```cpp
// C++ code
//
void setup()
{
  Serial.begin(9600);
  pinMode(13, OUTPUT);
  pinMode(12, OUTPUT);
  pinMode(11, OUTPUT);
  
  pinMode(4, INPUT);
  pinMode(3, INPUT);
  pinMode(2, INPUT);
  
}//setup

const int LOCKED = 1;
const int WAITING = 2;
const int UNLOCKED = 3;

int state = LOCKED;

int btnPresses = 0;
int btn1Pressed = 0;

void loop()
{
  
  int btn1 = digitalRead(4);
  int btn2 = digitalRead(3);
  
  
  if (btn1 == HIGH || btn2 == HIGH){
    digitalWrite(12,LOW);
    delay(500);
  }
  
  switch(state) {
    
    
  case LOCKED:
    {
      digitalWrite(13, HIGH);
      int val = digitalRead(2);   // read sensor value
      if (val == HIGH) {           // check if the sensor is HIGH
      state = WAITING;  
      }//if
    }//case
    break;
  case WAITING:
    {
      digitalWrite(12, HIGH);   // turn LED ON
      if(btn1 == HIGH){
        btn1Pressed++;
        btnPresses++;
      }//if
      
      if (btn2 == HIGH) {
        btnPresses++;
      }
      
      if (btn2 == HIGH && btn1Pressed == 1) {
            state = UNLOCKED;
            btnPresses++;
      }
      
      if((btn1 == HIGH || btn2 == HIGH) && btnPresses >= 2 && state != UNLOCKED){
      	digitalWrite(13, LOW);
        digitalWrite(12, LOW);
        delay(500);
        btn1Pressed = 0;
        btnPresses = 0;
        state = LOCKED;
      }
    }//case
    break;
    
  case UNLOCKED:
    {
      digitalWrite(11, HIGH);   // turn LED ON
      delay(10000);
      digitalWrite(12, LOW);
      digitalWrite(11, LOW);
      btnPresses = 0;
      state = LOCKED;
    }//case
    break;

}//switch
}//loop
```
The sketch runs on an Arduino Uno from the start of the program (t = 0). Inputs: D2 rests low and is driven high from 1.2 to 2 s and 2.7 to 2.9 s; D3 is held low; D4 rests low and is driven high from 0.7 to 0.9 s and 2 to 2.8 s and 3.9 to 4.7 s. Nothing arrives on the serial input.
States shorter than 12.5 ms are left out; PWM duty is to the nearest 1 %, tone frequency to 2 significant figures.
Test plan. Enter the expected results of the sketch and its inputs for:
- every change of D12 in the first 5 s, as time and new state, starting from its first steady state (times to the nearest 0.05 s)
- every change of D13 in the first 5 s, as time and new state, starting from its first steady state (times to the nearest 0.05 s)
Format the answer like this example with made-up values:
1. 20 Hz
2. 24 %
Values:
1. 0 s low; 1.2 s high; 2 s low
2. 0 s high; 3 s low; 3.5 s high
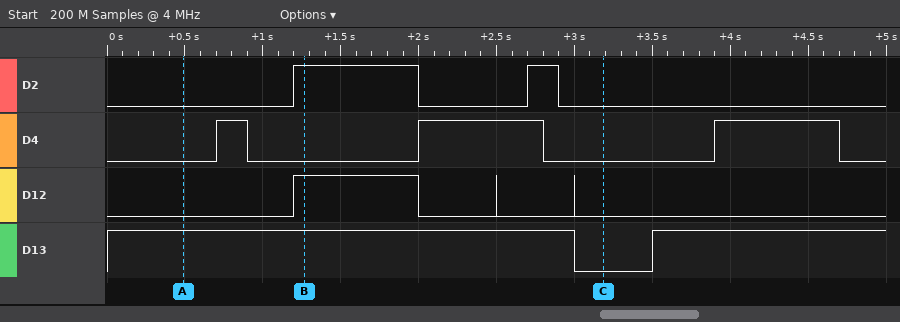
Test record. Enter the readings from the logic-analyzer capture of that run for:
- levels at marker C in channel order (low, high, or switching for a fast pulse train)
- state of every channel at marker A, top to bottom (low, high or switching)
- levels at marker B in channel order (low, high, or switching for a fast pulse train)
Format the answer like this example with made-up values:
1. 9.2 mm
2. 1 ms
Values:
1. D2 low, D4 low, D12 low, D13 low
2. D2 low, D4 low, D12 low, D13 high
3. D2 high, D4 low, D12 high, D13 high
